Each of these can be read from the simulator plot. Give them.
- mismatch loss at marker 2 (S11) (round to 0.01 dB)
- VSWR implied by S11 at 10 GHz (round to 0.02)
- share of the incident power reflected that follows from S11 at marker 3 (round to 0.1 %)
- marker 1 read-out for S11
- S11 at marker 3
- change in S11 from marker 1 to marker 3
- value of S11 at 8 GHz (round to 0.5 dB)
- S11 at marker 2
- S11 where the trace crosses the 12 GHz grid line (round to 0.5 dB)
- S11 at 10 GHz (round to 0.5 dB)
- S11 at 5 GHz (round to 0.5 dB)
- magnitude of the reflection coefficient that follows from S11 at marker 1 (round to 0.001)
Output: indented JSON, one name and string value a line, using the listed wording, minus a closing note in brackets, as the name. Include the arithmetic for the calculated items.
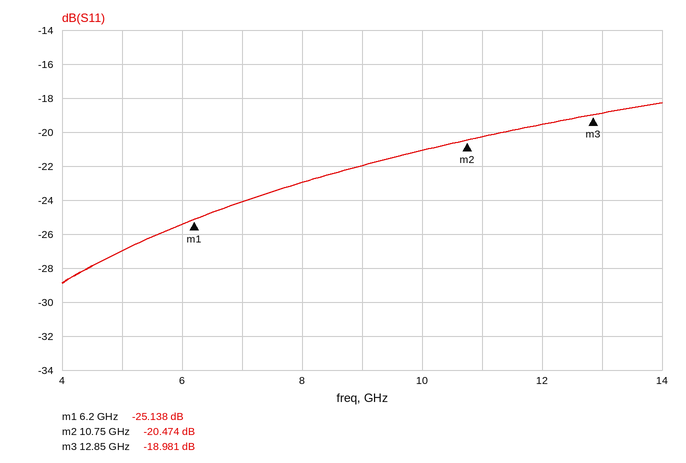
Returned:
{
  "mismatch loss at marker 2 (S11)": "−10 log10(1 − 10^(-20.474/10)) ≈ 0.04 dB",
  "VSWR implied by S11 at 10 GHz": "|Γ| = 10^(-21/20) = 0.0891; VSWR = (1 + 0.0891)/(1 − 0.0891) ≈ 1.20",
  "share of the incident power reflected that follows from S11 at marker 3": "10^(-18.981/10) ≈ 1.3 %",
  "marker 1 read-out for S11": "-25.138 dB",
  "S11 at marker 3": "-18.981 dB",
  "change in S11 from marker 1 to marker 3": "-18.981 − (-25.138) = 6.157 dB",
  "value of S11 at 8 GHz": "-23.0 dB",
  "S11 at marker 2": "-20.474 dB",
  "S11 where the trace crosses the 12 GHz grid line": "-19.5 dB",
  "S11 at 10 GHz": "-21.0 dB",
  "S11 at 5 GHz": "-27.0 dB",
  "magnitude of the reflection coefficient that follows from S11 at marker 1": "10^(-25.138/20) ≈ 0.055"
}
